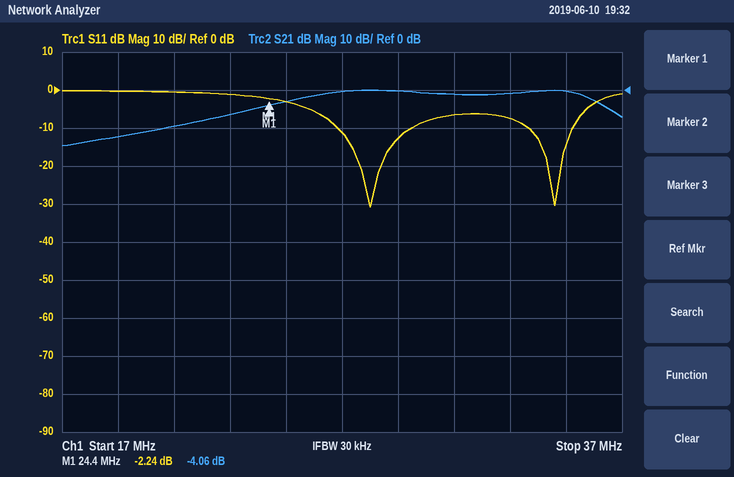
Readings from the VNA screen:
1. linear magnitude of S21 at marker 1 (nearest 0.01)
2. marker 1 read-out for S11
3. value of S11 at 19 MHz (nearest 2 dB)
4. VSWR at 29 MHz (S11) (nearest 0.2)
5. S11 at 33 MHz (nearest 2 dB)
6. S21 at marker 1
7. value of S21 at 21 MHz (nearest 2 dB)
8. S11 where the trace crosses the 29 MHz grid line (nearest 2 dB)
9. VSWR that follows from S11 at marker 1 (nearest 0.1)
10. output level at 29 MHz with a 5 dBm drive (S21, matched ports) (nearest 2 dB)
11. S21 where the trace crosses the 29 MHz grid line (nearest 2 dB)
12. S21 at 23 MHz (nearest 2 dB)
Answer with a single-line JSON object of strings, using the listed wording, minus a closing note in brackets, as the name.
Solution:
{"linear magnitude of S21 at marker 1": "0.63", "marker 1 read-out for S11": "-2.24 dB", "value of S11 at 19 MHz": "0 dB", "VSWR at 29 MHz (S11)": "1.6", "S11 at 33 MHz": "-8 dB", "S21 at marker 1": "-4.06 dB", "value of S21 at 21 MHz": "-10 dB", "S11 where the trace crosses the 29 MHz grid line": "-12 dB", "VSWR that follows from S11 at marker 1": "7.8", "output level at 29 MHz with a 5 dBm drive (S21, matched ports)": "4 dBm", "S21 where the trace crosses the 29 MHz grid line": "0 dB", "S21 at 23 MHz": "-6 dB"}
